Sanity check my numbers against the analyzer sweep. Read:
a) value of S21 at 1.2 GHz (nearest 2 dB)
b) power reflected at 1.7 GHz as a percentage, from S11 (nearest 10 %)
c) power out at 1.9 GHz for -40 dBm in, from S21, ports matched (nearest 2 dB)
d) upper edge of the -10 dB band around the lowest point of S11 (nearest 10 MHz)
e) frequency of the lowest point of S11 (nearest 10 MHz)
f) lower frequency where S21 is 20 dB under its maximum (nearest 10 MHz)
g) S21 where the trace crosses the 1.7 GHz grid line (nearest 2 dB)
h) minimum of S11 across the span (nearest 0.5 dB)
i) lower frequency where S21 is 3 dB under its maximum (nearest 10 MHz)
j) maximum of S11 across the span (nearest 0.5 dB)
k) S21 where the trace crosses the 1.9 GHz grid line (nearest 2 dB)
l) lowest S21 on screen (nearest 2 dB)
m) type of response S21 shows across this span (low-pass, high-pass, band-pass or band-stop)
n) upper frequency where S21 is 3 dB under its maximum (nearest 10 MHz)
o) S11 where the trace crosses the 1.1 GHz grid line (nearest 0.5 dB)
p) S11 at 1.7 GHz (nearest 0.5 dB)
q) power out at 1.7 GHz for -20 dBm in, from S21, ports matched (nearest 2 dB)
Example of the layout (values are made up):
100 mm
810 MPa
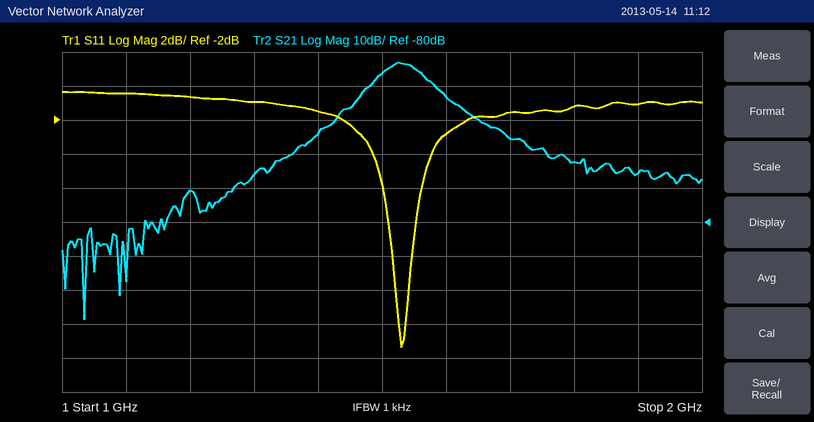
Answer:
-70 dB
70 %
-106 dBm
1.55 GHz
1.53 GHz
1.40 GHz
-56 dB
-15.5 dB
1.50 GHz
-0.5 dB
-66 dB
-108 dB
band-pass
1.56 GHz
-0.5 dB
-1.5 dB
-76 dBm
